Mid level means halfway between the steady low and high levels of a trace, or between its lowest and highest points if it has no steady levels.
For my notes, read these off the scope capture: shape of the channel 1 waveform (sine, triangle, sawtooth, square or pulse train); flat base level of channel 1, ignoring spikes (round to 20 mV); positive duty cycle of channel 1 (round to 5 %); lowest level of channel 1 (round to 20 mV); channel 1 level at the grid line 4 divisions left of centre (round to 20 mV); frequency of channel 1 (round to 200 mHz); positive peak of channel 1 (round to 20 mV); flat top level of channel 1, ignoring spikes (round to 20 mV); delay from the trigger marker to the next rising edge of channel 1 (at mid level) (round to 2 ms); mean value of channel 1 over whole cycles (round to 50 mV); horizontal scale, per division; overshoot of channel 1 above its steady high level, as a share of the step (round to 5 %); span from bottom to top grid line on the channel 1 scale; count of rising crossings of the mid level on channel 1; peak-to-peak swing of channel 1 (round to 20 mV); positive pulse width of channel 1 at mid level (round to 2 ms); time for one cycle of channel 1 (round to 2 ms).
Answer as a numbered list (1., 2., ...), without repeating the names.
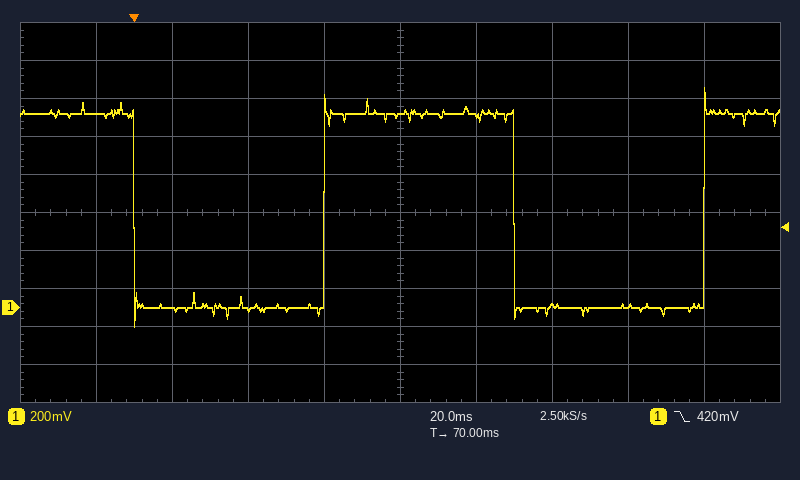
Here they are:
1. square
2. 0 mV
3. 50 %
4. -100 mV
5. 1.02 V
6. 10.0 Hz
7. 1.16 V
8. 1.02 V
9. 50 ms
10. 500 mV
11. 20 ms
12. 15 %
13. 2 V
14. 2
15. 1.26 V
16. 50 ms
17. 100 ms
